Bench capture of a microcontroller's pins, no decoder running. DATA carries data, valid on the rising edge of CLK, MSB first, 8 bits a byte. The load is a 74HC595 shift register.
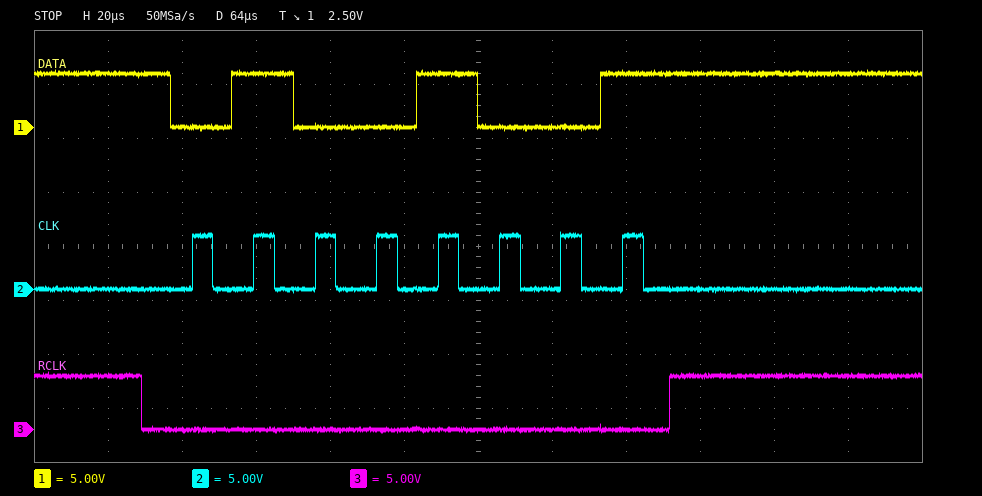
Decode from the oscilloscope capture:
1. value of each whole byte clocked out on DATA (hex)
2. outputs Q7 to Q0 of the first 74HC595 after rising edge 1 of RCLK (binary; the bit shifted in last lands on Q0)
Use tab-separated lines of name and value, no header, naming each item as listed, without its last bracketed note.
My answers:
value of each whole byte clocked out on DATA	49
outputs Q7 to Q0 of the first 74HC595 after rising edge 1 of RCLK	01001001
